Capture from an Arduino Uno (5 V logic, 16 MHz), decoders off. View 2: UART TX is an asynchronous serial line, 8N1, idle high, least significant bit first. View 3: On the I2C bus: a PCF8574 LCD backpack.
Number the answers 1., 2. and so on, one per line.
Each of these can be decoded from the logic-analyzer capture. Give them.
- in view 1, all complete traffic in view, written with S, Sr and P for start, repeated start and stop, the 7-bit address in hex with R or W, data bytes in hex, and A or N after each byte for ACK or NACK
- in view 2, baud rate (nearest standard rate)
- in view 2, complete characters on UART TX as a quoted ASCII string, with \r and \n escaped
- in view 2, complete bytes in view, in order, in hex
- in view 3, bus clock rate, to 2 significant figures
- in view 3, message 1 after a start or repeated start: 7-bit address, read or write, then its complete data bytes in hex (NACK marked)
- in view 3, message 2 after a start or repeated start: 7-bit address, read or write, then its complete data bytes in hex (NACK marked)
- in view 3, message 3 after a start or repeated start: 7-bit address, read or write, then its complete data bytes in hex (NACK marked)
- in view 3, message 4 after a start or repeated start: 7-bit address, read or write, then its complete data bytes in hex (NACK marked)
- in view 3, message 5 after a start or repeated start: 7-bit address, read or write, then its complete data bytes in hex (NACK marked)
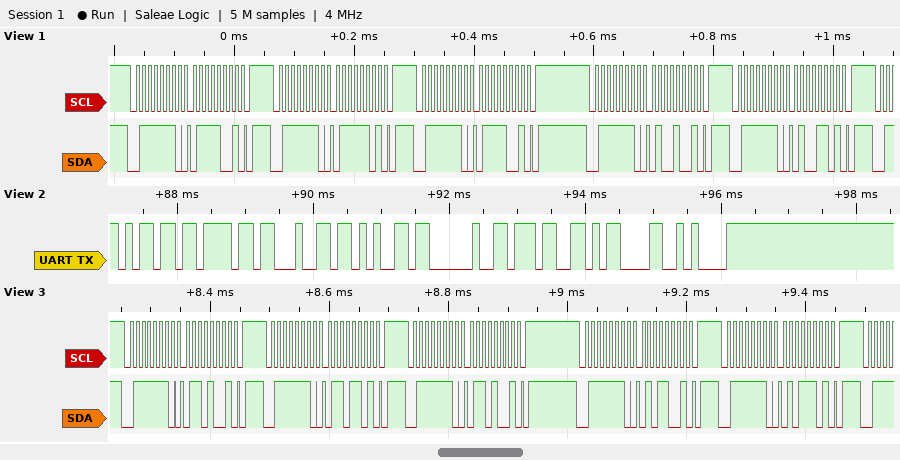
1. S 3FW A 79 A P S 3FW A 7D A P S 3FW A 79 A P S 3FW A 49 A P S 3FW A 4D A P
2. 9600 baud
3. "mode 7\r\n"
4. 6D 6F 64 65 20 37 0D 0A
5. 100 kHz
6. 0x3F write: 69
7. 0x3F write: 6D
8. 0x3F write: 69
9. 0x3F write: 59
10. 0x3F write: 5D
